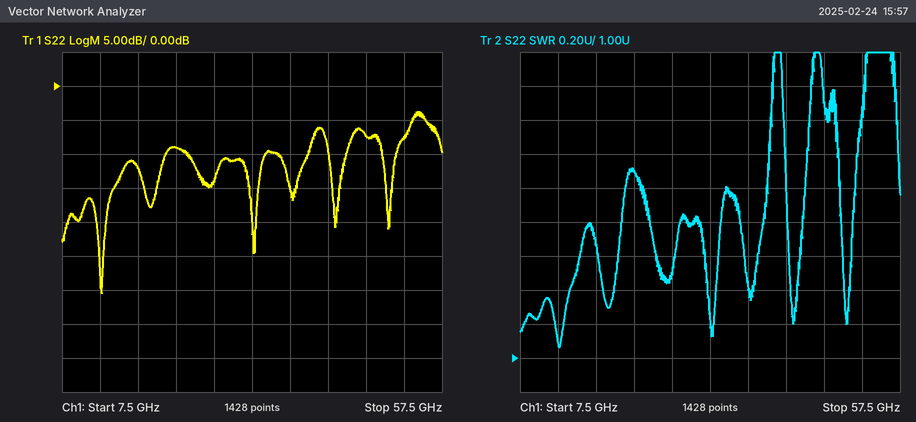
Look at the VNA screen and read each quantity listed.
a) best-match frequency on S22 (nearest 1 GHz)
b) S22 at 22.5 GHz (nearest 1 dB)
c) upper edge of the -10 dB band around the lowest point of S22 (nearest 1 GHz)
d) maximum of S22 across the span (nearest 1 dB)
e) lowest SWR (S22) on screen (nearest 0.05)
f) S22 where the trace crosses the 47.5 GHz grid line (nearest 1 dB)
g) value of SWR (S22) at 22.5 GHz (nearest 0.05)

13 GHz
-9 dB
21 GHz
-4 dB
1.05
-7 dB
2.10
